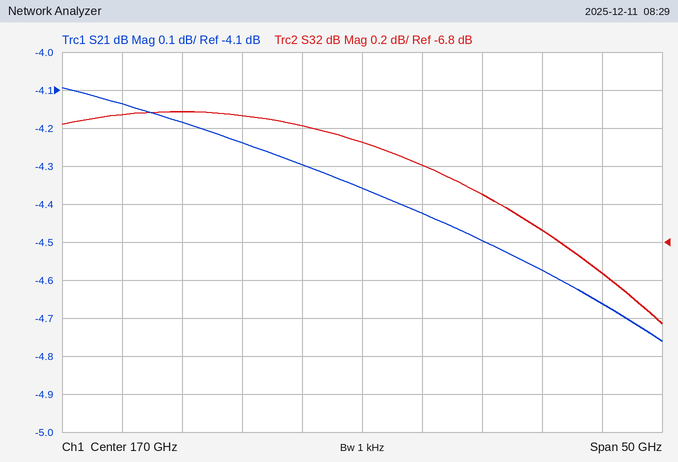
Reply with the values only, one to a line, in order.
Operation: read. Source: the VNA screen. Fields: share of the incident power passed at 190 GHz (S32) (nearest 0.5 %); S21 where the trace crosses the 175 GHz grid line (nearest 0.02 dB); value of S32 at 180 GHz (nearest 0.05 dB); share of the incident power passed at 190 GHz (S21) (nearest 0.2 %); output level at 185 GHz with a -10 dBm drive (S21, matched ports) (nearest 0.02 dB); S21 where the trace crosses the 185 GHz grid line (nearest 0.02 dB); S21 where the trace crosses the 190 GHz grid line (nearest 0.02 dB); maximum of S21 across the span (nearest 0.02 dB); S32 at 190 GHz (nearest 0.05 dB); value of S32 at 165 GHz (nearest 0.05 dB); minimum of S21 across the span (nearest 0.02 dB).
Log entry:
20.0 %
-4.42 dB
-6.55 dB
34.2 %
-14.58 dBm
-4.58 dB
-4.66 dB
-4.10 dB
-6.95 dB
-6.20 dB
-4.76 dB
